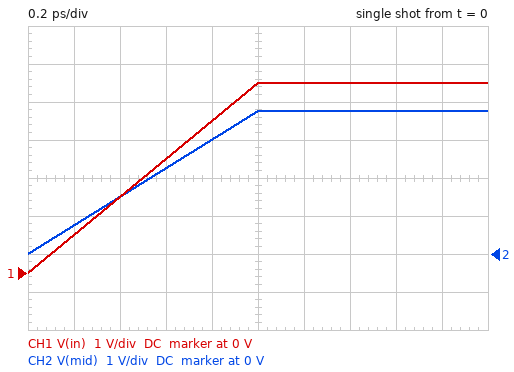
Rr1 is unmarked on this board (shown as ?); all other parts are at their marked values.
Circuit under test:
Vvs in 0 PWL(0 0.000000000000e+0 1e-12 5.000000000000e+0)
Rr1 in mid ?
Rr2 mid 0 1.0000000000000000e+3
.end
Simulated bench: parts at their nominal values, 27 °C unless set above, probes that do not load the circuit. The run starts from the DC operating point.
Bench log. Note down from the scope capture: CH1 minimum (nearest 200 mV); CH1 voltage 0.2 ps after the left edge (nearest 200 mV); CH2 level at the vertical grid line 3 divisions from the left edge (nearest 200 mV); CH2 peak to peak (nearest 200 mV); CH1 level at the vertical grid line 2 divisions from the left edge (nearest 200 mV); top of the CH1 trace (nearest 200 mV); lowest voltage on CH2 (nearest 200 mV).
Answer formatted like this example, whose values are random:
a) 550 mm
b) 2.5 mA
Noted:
a) 0 V
b) 1.0 V
c) 2.2 V
d) 3.8 V
e) 2.0 V
f) 5.0 V
g) 0 V
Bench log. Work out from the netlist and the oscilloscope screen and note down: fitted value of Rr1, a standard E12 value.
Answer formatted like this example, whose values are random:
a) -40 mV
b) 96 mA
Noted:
a) 330 Ω
